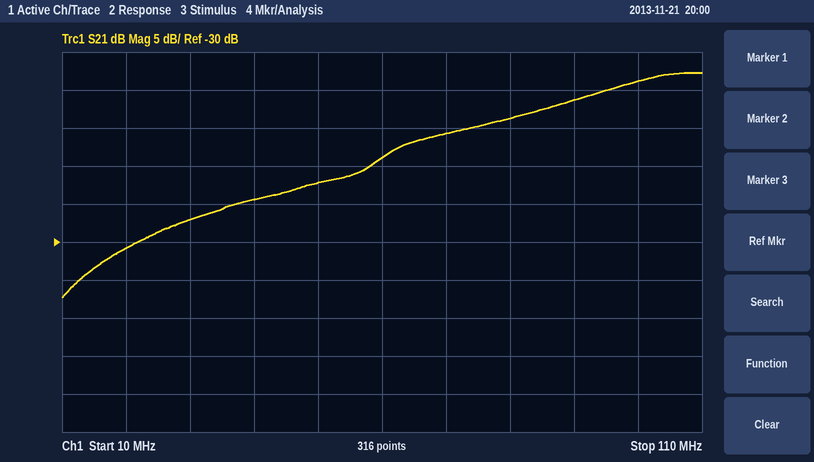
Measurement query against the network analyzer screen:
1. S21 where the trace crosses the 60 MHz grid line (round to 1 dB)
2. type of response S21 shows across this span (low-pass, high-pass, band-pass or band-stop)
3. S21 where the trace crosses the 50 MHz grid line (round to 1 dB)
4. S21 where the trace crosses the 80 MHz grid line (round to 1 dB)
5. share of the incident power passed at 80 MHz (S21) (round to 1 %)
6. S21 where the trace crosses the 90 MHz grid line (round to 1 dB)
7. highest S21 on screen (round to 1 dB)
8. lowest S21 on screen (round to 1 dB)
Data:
-19 dB
high-pass
-22 dB
-14 dB
4 %
-11 dB
-8 dB
-37 dB
